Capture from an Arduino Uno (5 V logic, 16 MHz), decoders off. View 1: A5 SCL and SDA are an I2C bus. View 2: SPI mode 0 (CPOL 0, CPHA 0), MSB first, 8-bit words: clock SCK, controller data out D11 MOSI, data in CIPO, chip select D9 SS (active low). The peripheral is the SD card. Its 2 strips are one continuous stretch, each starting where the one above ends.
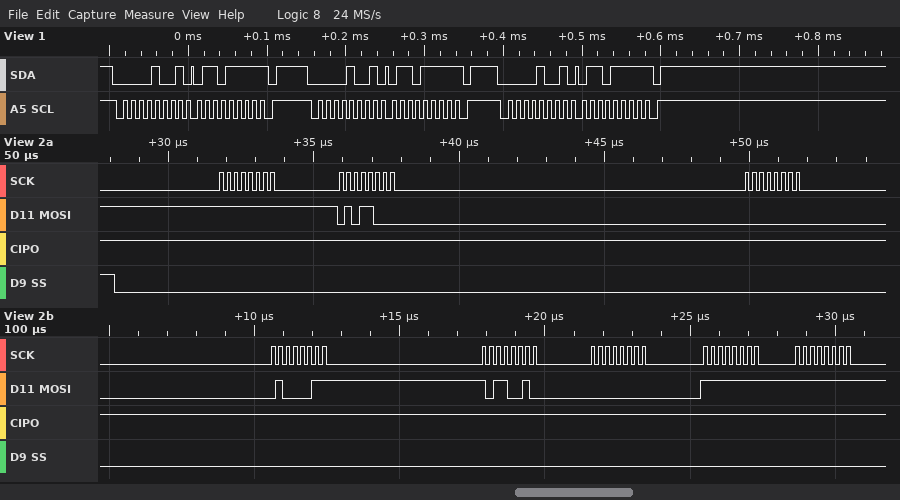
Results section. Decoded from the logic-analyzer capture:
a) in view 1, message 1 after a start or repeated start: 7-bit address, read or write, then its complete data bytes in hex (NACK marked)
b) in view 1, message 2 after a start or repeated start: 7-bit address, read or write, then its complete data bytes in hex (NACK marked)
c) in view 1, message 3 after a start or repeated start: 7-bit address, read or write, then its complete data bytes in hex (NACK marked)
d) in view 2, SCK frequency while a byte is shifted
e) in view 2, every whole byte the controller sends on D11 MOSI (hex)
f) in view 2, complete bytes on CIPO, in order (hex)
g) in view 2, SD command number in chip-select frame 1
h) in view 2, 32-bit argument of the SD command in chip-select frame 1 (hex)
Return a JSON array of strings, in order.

["0x04 read: 6F NACK", "0x04 read: 6F NACK", "0x04 read: 6F NACK", "4 MHz", "0xFF 0x58 0x00 0x43 0xB2 0x00 0xFF 0xFF", "0xFF 0xFF 0xFF 0xFF 0xFF 0xFF 0xFF 0xFF", "CMD24", "0x0043B200"]
